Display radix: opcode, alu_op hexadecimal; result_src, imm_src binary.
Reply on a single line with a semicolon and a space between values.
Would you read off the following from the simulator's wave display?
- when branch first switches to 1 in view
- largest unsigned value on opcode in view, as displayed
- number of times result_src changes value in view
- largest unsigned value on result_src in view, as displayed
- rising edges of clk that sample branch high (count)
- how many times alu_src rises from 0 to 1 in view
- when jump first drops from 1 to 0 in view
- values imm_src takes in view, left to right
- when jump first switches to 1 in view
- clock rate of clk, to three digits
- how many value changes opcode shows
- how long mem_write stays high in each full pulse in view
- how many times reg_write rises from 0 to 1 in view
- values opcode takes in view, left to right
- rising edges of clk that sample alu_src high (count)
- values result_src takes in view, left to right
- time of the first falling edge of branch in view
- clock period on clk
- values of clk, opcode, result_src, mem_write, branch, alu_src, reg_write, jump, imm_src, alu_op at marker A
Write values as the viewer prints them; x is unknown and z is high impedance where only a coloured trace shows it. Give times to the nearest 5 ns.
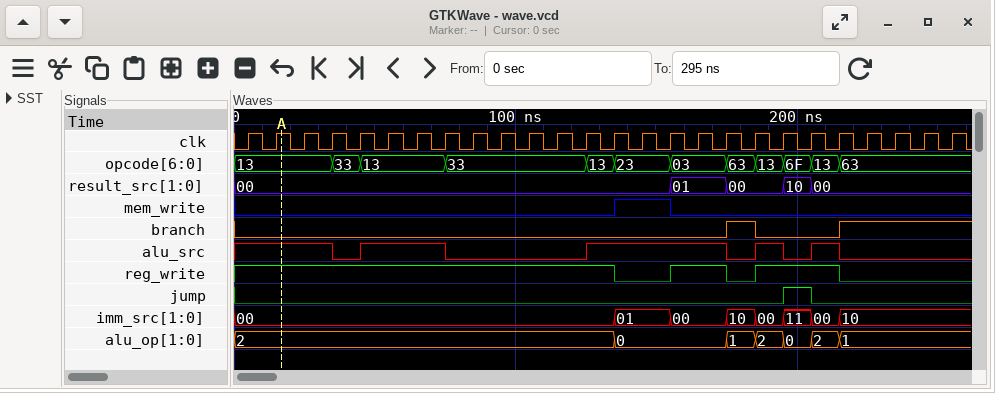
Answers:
175 ns; 6F; 4; 10; 5; 4; 205 ns; 00, 01, 00, 10, 00, 11, 00, 10; 195 ns; 100 MHz; 11; 20 ns; 2; 13, 33, 13, 33, 13, 23, 03, 63, 13, 6F, 13, 63; 14; 00, 01, 00, 10, 00; 185 ns; 10 ns; clk=1, opcode=13, result_src=00, mem_write=0, branch=0, alu_src=1, reg_write=1, jump=0, imm_src=00, alu_op=2
